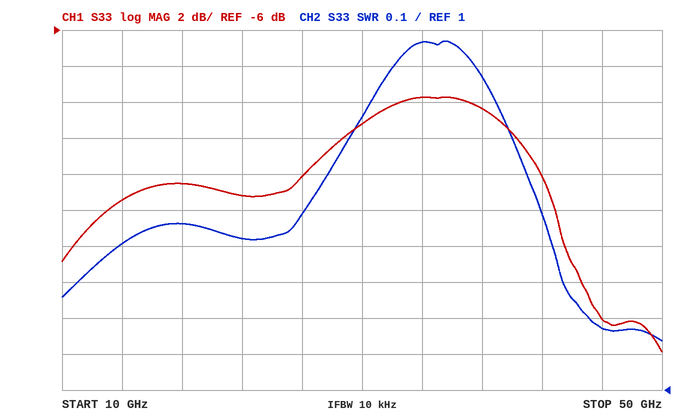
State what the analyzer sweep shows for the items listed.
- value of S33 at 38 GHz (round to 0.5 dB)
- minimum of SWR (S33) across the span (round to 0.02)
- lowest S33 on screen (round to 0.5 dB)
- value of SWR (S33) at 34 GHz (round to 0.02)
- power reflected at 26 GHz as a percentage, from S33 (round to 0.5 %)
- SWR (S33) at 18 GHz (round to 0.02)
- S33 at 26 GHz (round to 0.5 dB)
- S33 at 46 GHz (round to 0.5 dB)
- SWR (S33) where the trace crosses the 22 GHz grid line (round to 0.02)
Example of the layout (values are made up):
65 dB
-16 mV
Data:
-10.5 dB
1.14
-24.0 dB
1.96
4.0 %
1.46
-14.0 dB
-22.0 dB
1.42
